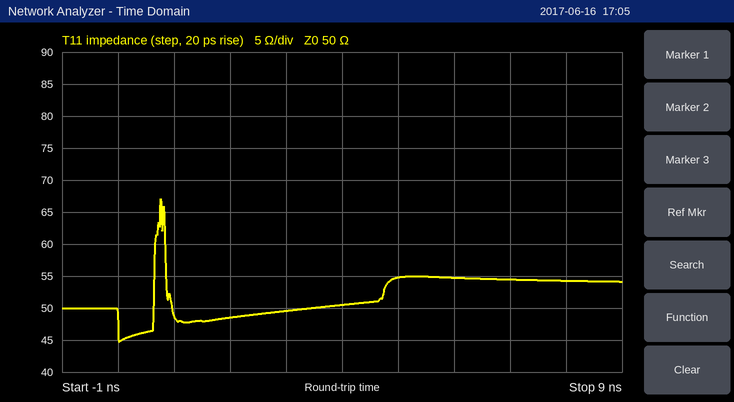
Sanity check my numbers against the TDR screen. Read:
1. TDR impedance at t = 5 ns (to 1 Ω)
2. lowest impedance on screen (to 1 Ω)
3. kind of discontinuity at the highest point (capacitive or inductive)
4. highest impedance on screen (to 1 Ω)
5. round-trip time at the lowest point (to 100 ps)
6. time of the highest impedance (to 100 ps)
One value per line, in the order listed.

55 Ω
45 Ω
inductive
67 Ω
0.0 ns
800 ps
